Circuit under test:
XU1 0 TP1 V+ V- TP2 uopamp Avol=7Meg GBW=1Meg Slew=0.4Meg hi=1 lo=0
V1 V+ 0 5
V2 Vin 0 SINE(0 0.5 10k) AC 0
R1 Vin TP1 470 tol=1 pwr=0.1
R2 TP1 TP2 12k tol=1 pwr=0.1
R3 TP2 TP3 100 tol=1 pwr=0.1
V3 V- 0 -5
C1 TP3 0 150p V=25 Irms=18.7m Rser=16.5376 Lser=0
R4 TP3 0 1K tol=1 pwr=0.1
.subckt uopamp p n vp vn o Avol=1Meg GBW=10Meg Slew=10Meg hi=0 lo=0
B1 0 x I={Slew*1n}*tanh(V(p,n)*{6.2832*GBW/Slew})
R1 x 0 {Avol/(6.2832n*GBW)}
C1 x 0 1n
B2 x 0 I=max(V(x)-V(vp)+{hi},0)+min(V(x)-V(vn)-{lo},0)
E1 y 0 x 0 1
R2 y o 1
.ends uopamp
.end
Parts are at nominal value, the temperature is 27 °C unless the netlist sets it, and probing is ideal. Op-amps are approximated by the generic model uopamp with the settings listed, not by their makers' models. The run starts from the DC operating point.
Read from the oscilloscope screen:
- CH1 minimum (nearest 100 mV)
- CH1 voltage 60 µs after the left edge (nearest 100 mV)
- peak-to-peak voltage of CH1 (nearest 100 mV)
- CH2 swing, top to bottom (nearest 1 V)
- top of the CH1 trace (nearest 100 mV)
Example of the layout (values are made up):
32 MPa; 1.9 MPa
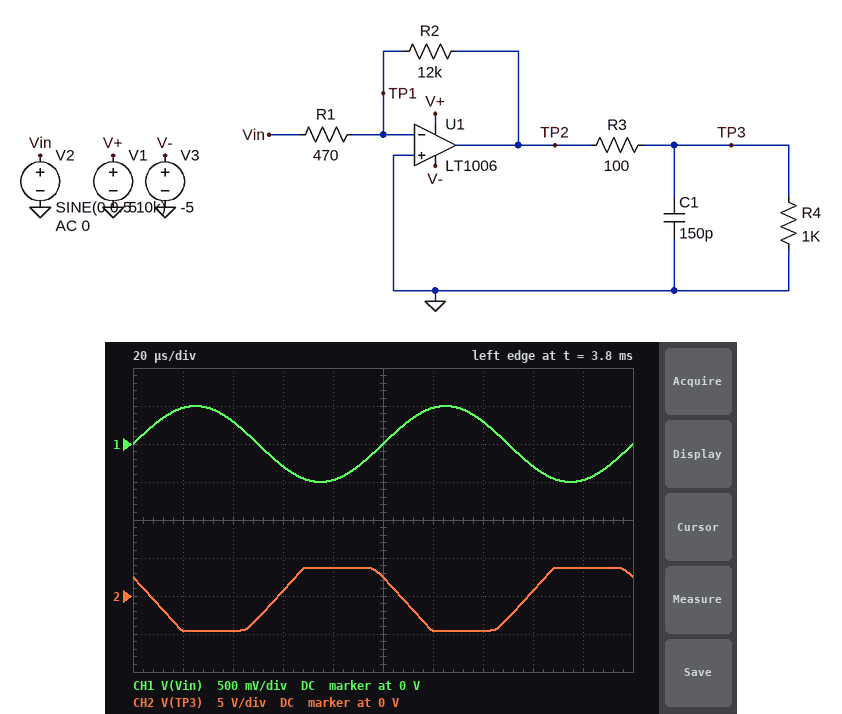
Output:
-500 mV; -300 mV; 1.0 V; 8 V; 500 mV
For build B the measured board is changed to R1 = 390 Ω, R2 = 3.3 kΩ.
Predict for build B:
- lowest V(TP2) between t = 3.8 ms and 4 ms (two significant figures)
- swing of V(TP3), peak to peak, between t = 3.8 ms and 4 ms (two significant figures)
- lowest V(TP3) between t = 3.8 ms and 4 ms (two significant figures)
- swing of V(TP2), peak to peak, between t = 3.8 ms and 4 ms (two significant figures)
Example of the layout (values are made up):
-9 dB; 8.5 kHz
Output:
-4.2 V; 7.5 V; -3.8 V; 8.2 V
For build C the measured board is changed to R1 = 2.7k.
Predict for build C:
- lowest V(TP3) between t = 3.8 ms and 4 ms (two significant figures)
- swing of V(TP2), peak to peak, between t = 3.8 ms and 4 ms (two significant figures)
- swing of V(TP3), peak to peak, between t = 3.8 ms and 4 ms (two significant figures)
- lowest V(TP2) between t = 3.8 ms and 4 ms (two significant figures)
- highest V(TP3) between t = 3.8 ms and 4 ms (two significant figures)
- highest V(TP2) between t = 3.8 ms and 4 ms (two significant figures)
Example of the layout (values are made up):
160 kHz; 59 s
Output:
-2.0 V; 4.4 V; 4.0 V; -2.2 V; 2.0 V; 2.2 V
